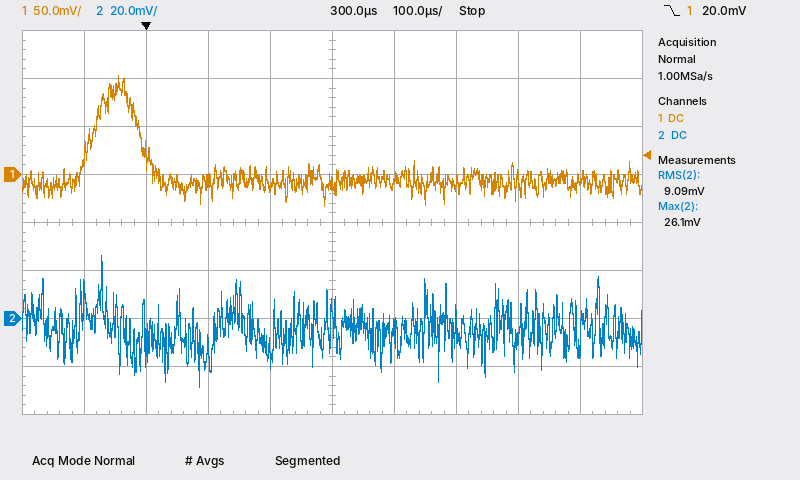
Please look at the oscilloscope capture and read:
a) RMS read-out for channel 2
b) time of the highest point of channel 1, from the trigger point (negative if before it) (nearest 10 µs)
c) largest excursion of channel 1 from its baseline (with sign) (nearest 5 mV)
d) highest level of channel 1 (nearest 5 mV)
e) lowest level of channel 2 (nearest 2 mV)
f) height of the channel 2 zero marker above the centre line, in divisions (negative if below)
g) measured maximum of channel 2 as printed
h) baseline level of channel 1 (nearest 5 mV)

9.09 mV
-40 µs
+110 mV
105 mV
-28 mV
-2.0 div
26.1 mV
-5 mV
